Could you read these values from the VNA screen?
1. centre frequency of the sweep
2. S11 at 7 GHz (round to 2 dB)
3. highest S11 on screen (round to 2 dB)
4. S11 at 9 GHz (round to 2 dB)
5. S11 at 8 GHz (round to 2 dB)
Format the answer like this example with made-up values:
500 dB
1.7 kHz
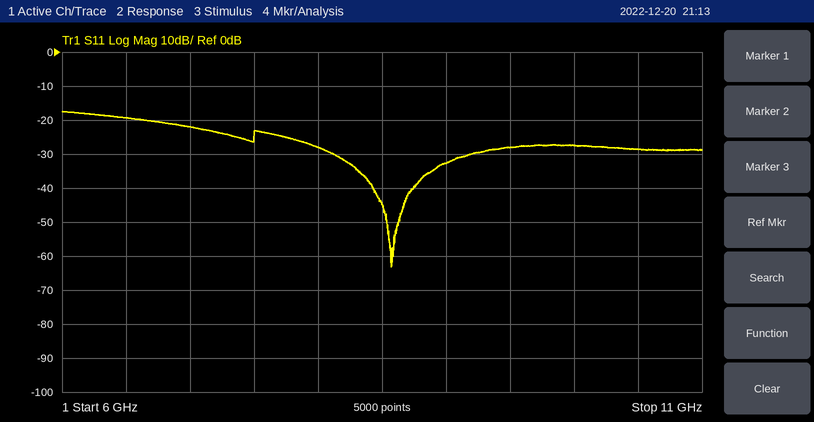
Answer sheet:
8.5 GHz
-22 dB
-18 dB
-32 dB
-28 dB
